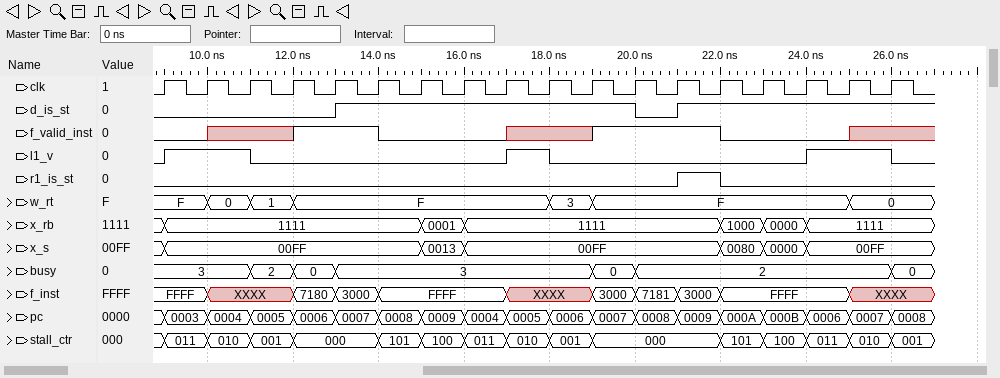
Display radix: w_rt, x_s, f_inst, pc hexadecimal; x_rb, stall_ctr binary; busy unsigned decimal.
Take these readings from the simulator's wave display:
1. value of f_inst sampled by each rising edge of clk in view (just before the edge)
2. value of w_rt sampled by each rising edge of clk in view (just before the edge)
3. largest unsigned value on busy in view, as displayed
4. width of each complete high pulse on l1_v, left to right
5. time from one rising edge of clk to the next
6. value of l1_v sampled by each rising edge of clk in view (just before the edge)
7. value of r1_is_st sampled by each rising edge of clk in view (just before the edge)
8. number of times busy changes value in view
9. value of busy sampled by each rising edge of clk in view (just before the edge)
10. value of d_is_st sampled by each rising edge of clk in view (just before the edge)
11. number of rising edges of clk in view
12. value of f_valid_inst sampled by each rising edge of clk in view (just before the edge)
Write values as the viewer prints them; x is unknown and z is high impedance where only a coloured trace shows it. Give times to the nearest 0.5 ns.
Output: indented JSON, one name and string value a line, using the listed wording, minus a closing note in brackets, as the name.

{
  "value of f_inst sampled by each rising edge of clk in view": "FFFF, FFFF, XXXX, XXXX, 7180, 3000, FFFF, FFFF, FFFF, XXXX, XXXX, 3000, 7181, 3000, FFFF, FFFF, FFFF, XXXX",
  "value of w_rt sampled by each rising edge of clk in view": "F, F, 0, 1, F, F, F, F, F, F, 3, F, F, F, F, F, F, 0",
  "largest unsigned value on busy in view, as displayed": "3",
  "width of each complete high pulse on l1_v, left to right": "2 ns, 1 ns, 2 ns",
  "time from one rising edge of clk to the next": "1 ns",
  "value of l1_v sampled by each rising edge of clk in view": "0 1 1 0 0 0 0 0 0 1 0 0 0 0 0 0 1 1",
  "value of r1_is_st sampled by each rising edge of clk in view": "0 0 0 0 0 0 0 0 0 0 0 0 0 1 0 0 0 0",
  "number of times busy changes value in view": "6",
  "value of busy sampled by each rising edge of clk in view": "3, 3, 3, 2, 0, 3, 3, 3, 3, 3, 3, 0, 2, 2, 2, 2, 2, 2",
  "value of d_is_st sampled by each rising edge of clk in view": "0 0 0 0 0 1 1 1 1 1 1 1 0 1 1 1 1 1",
  "number of rising edges of clk in view": "18",
  "value of f_valid_inst sampled by each rising edge of clk in view": "0 0 x x 1 1 0 0 0 x x 1 1 1 0 0 0 x"
}
